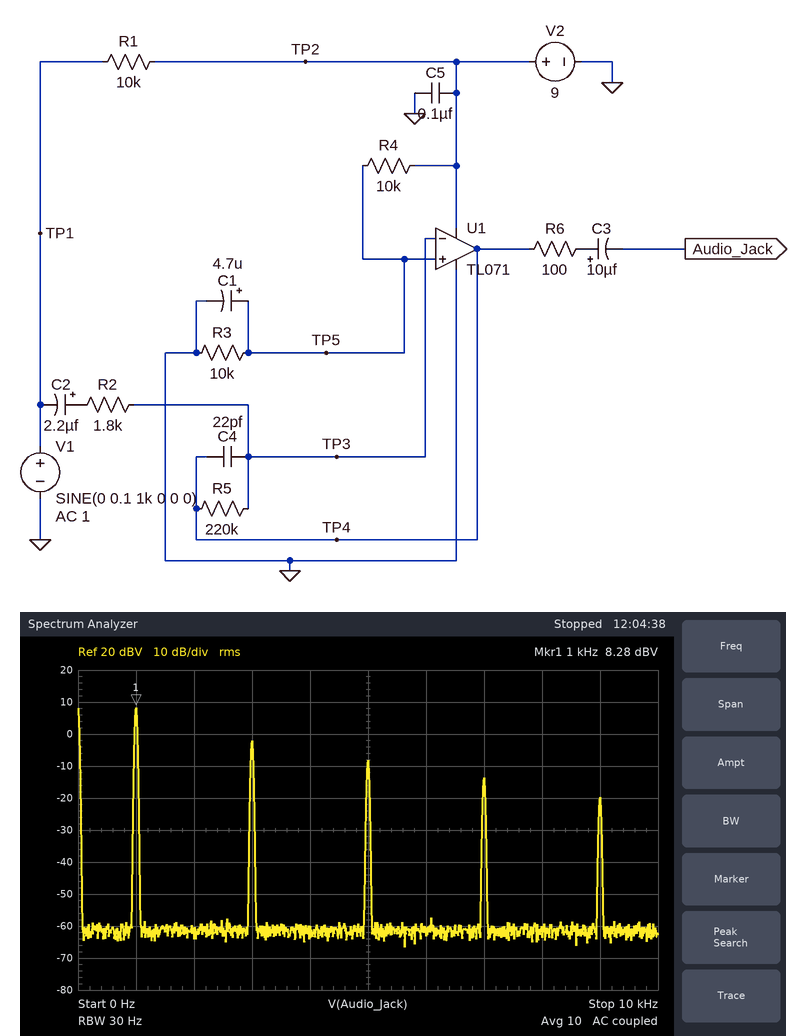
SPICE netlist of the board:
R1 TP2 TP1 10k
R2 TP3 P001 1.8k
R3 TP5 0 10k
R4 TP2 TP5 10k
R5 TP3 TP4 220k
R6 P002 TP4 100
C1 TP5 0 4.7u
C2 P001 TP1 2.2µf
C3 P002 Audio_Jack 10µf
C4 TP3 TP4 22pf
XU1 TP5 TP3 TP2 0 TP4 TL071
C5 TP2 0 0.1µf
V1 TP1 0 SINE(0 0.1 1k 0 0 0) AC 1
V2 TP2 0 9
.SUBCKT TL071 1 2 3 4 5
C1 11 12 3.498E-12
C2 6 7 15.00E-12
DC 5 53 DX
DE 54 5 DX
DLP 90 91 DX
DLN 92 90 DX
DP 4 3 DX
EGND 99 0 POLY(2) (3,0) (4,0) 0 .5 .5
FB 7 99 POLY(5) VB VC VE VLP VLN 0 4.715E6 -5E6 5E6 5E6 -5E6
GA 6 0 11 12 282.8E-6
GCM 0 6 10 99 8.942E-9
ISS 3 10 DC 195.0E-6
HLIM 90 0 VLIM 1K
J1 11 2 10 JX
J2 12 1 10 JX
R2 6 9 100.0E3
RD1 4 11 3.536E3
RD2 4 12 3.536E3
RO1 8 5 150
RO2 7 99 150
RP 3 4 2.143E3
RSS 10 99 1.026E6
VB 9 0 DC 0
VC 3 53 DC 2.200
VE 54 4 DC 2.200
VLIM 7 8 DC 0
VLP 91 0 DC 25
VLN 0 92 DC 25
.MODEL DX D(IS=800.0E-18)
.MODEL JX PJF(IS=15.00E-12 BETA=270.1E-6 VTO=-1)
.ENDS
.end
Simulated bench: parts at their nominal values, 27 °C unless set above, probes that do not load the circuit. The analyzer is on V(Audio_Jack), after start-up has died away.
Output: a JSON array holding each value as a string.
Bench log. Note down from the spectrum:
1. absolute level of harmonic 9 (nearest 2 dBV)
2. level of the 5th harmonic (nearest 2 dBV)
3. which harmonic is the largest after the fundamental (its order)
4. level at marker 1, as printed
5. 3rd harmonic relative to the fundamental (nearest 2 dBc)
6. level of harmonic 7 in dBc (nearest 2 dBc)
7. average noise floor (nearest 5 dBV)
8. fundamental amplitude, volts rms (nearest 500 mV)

["-20 dBV", "-8 dBV", "3", "8.28 dBV", "-10 dBc", "-22 dBc", "-60 dBV", "2.5 V"]
